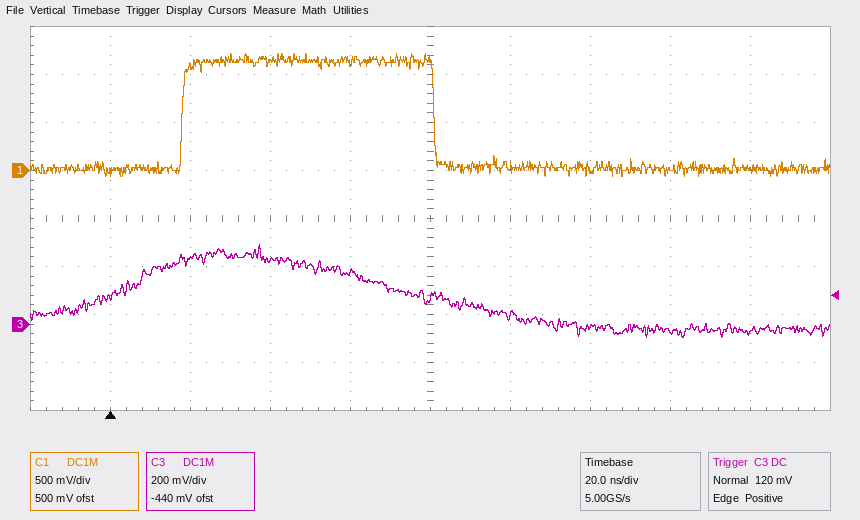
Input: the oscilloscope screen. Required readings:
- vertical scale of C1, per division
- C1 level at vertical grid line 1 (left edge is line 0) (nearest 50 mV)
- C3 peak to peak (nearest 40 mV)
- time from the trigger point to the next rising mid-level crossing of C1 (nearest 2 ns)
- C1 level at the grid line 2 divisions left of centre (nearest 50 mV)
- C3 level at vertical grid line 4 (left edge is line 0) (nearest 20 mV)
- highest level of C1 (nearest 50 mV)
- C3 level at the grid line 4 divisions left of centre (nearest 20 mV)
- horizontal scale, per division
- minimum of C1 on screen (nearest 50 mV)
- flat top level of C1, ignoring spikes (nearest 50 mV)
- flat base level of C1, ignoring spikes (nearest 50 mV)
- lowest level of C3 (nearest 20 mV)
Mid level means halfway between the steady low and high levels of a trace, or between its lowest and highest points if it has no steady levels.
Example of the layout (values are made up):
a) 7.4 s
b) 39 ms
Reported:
a) 500 mV
b) 0 mV
c) 400 mV
d) 18 ns
e) 1.15 V
f) 220 mV
g) 1.20 V
h) 120 mV
i) 20 ns
j) -50 mV
k) 1.15 V
l) 0 mV
m) -60 mV
